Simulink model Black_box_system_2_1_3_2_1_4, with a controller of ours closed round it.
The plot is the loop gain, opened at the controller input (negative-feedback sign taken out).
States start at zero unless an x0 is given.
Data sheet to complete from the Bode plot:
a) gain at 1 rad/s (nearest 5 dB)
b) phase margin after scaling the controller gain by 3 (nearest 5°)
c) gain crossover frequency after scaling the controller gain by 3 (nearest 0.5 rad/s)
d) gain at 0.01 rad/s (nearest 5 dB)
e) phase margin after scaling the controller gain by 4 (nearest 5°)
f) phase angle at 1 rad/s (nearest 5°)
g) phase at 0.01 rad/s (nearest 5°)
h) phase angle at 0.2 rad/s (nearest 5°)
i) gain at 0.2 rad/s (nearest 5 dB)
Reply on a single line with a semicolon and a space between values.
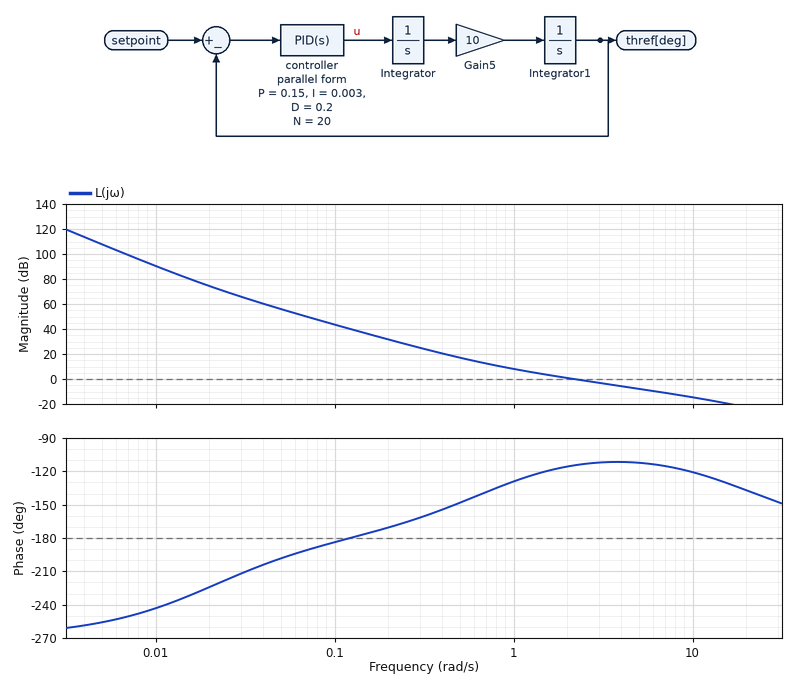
10 dB; 65°; 6.0 rad/s; 90 dB; 65°; -130°; -245°; -170°; 30 dB
